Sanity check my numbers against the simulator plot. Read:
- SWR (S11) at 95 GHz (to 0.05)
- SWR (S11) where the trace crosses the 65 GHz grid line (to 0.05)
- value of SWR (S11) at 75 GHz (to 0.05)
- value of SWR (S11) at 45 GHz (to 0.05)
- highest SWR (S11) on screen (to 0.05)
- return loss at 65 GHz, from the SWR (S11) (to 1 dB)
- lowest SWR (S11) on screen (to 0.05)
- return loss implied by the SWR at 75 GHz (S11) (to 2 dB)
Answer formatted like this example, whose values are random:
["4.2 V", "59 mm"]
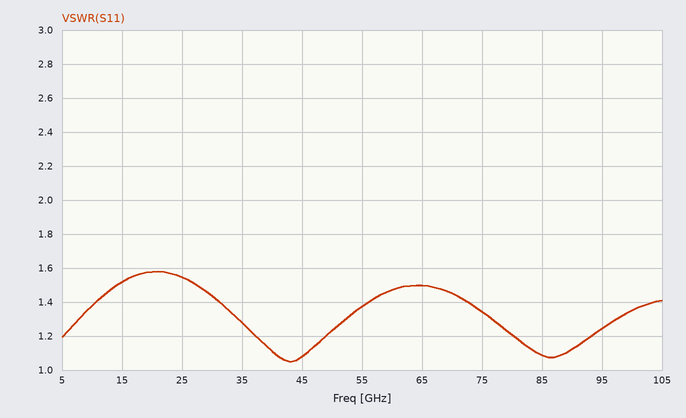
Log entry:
["1.25", "1.50", "1.35", "1.10", "1.60", "14 dB", "1.05", "16 dB"]
